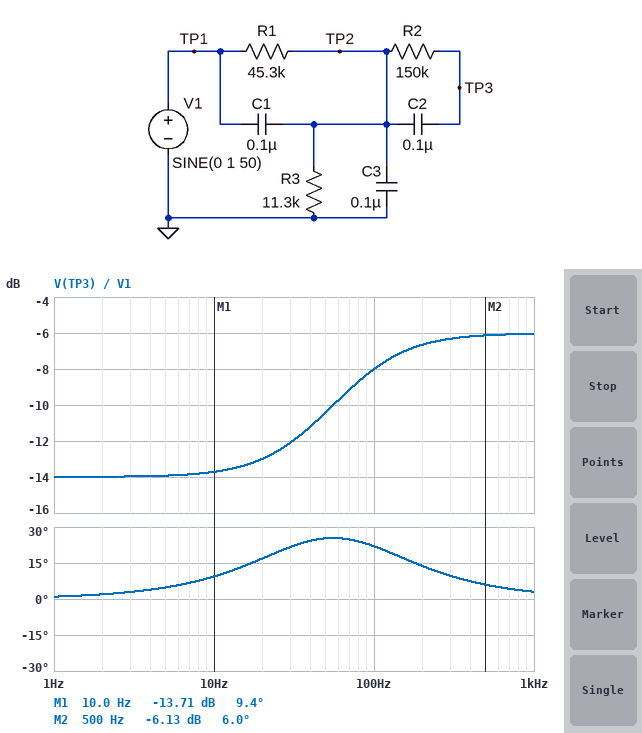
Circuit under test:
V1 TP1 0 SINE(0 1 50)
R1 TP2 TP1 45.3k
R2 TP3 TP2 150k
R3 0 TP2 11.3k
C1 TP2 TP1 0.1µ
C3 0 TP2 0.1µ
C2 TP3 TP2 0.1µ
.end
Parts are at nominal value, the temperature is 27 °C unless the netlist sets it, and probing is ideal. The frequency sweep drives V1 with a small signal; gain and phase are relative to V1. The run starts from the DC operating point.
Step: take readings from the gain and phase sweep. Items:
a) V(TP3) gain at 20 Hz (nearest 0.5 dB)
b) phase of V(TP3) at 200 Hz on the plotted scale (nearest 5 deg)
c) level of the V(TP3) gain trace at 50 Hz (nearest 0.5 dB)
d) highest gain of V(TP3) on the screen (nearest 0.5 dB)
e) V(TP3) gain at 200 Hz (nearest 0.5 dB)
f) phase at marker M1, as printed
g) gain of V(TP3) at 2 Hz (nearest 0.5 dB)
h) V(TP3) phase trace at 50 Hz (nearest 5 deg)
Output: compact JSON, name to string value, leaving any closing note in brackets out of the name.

{"V(TP3) gain at 20 Hz": "-13.0 dB", "phase of V(TP3) at 200 Hz on the plotted scale": "15 deg", "level of the V(TP3) gain trace at 50 Hz": "-10.5 dB", "highest gain of V(TP3) on the screen": "-6.0 dB", "V(TP3) gain at 200 Hz": "-6.5 dB", "phase at marker M1, as printed": "9.4 deg", "gain of V(TP3) at 2 Hz": "-14.0 dB", "V(TP3) phase trace at 50 Hz": "25 deg"}
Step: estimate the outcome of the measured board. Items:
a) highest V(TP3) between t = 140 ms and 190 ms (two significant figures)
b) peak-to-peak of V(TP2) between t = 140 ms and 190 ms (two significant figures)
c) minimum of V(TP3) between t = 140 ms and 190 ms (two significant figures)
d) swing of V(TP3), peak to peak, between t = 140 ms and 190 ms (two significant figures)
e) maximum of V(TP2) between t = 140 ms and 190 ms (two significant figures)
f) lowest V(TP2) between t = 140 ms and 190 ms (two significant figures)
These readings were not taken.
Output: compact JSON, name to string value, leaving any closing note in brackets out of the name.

{"highest V(TP3) between t = 140 ms and 190 ms": "300 mV", "peak-to-peak of V(TP2) between t = 140 ms and 190 ms": "600 mV", "minimum of V(TP3) between t = 140 ms and 190 ms": "-300 mV", "swing of V(TP3), peak to peak, between t = 140 ms and 190 ms": "600 mV", "maximum of V(TP2) between t = 140 ms and 190 ms": "300 mV", "lowest V(TP2) between t = 140 ms and 190 ms": "-300 mV"}
